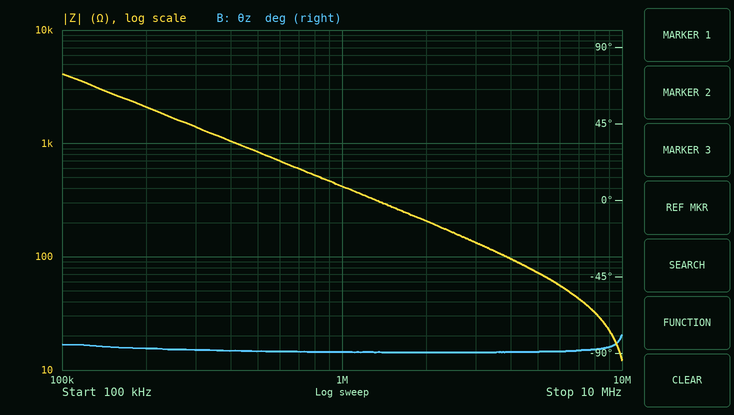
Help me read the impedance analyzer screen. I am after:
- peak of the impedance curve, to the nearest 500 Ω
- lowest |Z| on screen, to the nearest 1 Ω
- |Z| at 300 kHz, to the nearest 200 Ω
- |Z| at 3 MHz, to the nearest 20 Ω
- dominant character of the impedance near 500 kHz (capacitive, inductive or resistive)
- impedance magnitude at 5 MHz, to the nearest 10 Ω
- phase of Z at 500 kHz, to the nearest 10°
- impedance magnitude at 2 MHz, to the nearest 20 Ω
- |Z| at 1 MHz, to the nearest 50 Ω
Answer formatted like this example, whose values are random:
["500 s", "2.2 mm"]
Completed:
["4.0 kΩ", "12 Ω", "1.4 kΩ", "140 Ω", "capacitive", "70 Ω", "-90°", "200 Ω", "400 Ω"]
